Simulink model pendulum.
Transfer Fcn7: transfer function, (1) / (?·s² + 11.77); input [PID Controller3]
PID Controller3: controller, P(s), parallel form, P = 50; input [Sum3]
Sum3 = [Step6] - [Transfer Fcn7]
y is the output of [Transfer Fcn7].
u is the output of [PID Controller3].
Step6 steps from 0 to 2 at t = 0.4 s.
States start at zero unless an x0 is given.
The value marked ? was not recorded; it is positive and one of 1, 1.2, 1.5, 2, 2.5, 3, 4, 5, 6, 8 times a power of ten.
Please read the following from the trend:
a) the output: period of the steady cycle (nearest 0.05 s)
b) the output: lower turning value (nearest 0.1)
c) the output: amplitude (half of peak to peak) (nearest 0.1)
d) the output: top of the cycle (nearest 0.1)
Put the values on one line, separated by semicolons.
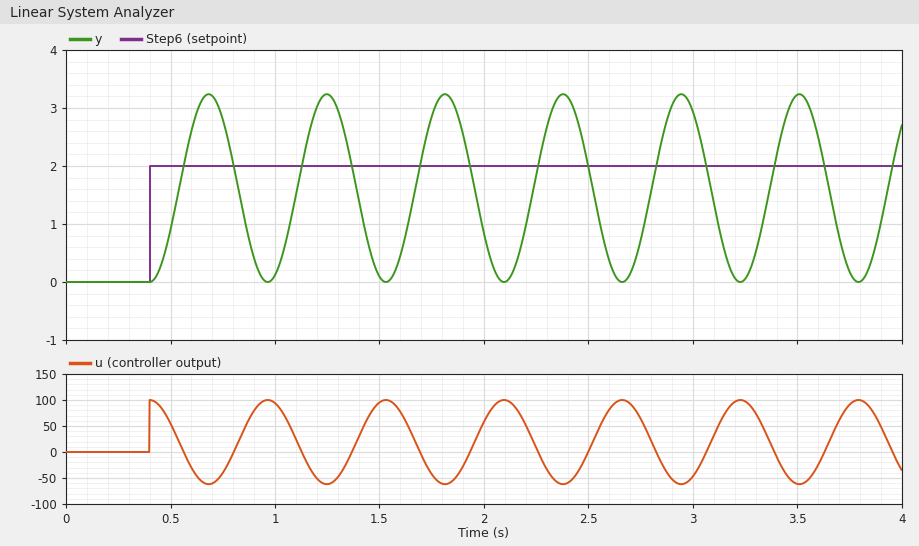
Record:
0.55 s; 0.0; 1.6; 3.2
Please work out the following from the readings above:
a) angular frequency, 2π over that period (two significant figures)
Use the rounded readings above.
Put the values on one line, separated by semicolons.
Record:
11 rad/s
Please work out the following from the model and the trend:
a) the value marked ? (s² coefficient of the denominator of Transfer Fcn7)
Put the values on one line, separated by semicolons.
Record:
0.5
